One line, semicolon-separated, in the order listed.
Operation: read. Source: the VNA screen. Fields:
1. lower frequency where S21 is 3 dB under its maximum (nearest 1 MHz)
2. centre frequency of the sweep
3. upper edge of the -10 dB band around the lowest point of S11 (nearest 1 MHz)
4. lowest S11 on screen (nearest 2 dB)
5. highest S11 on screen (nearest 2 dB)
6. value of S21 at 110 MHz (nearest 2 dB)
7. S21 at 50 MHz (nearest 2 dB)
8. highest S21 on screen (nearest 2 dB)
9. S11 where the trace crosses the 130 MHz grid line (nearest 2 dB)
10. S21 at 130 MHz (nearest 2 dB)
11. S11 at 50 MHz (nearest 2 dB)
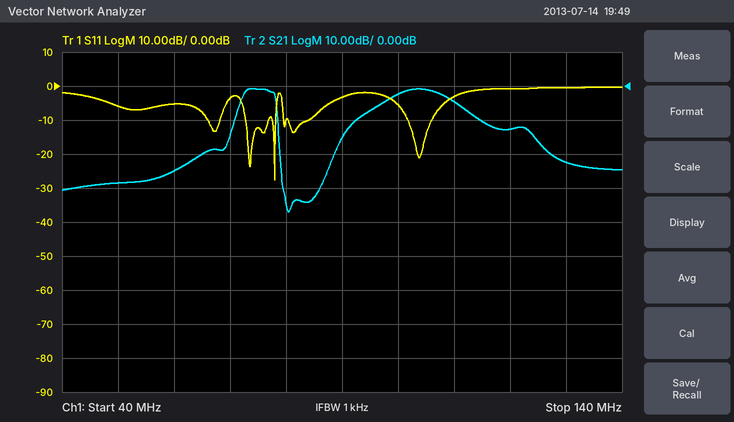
72 MHz; 90 MHz; 78 MHz; -28 dB; 0 dB; -4 dB; -28 dB; 0 dB; 0 dB; -22 dB; -6 dB
